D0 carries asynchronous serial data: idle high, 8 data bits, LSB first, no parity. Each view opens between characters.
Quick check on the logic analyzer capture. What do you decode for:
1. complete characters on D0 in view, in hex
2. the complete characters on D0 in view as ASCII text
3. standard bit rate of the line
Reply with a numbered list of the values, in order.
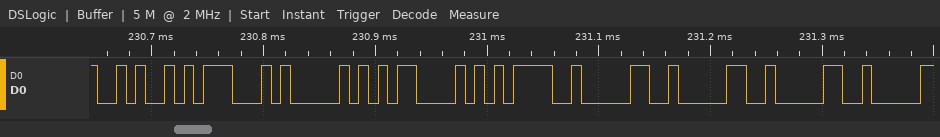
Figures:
1. 4A, 47, 50, 43, 3D, 30, 30, 30
2. "JGPC=000"
3. 115200 baud
